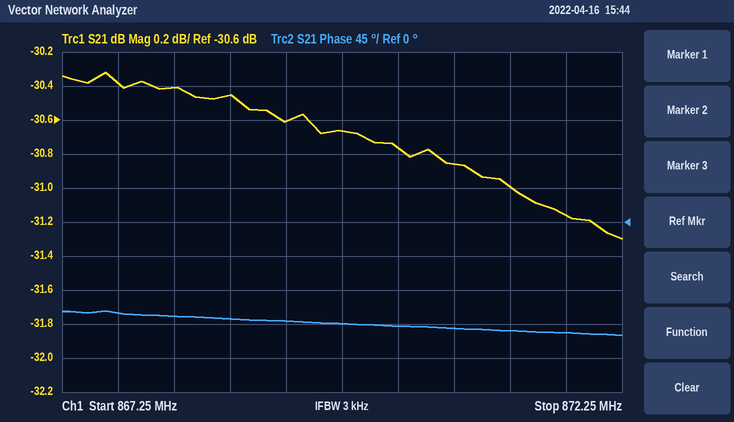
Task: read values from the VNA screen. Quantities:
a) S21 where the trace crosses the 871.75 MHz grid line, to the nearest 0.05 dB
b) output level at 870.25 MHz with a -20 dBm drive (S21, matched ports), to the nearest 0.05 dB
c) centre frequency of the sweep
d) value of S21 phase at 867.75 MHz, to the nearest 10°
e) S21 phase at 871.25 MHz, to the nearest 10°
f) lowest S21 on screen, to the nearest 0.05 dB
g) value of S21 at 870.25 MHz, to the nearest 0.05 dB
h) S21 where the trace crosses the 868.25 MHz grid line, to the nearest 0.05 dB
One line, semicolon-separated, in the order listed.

-31.15 dB; -50.75 dBm; 869.75 MHz; -120°; -140°; -31.30 dB; -30.75 dB; -30.40 dB
